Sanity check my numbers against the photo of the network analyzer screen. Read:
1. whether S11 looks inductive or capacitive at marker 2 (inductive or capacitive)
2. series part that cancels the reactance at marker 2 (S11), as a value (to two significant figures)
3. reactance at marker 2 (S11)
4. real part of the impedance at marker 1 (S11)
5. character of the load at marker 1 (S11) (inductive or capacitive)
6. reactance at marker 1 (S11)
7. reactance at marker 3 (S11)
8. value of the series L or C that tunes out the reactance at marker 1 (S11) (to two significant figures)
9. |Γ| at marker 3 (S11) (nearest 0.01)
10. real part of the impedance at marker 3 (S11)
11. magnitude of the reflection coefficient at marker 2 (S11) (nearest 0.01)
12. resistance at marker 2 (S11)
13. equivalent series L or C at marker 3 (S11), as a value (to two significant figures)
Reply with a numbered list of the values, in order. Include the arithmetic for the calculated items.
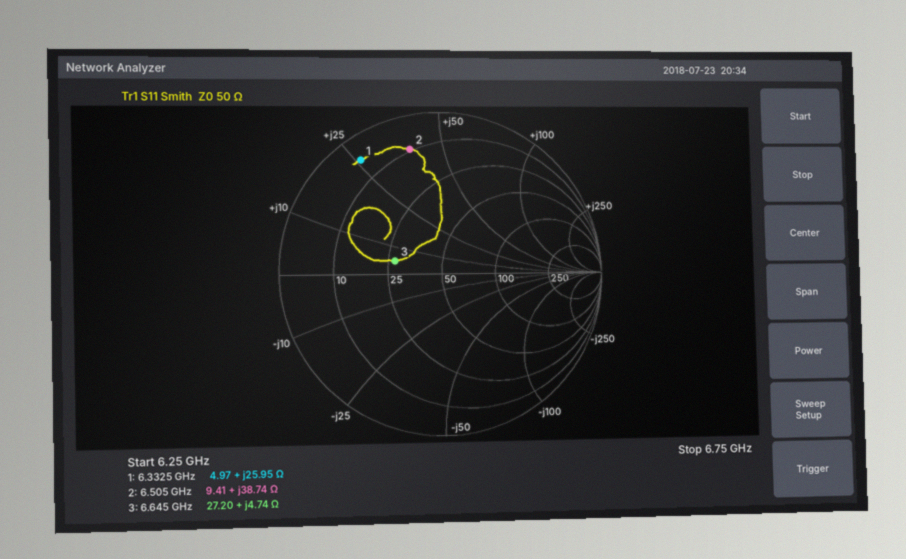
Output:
1. inductive
2. C = 1/(2π × 6.505 GHz × 38.74 Ω) ≈ 632 fF, so 630 fF to two significant figures
3. +38.74 Ω
4. 4.97 Ω
5. inductive
6. +25.95 Ω
7. +4.74 Ω
8. C = 1/(2π × 6.3325 GHz × 25.95 Ω) ≈ 969 fF, so 970 fF to two significant figures
9. 0.30
10. 27.20 Ω
11. 0.79
12. 9.41 Ω
13. L = 4.74 Ω/(2π × 6.645 GHz) ≈ 114 pH, so 110 pH to two significant figures
